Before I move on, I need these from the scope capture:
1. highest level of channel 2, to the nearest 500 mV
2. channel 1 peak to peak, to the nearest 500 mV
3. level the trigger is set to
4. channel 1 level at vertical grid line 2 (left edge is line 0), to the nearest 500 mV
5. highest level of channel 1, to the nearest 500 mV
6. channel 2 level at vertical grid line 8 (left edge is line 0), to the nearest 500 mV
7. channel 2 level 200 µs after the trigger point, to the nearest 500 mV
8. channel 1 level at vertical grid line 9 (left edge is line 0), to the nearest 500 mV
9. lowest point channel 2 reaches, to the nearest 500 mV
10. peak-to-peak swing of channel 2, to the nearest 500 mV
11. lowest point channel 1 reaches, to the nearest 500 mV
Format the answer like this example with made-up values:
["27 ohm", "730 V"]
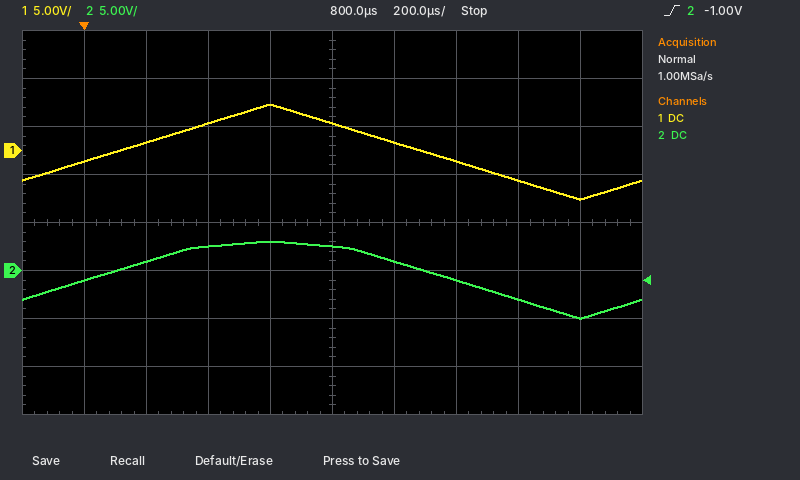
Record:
["3.0 V", "10.0 V", "-1.00 V", "1.0 V", "5.0 V", "-3.0 V", "1.0 V", "-5.0 V", "-5.0 V", "8.0 V", "-5.0 V"]
